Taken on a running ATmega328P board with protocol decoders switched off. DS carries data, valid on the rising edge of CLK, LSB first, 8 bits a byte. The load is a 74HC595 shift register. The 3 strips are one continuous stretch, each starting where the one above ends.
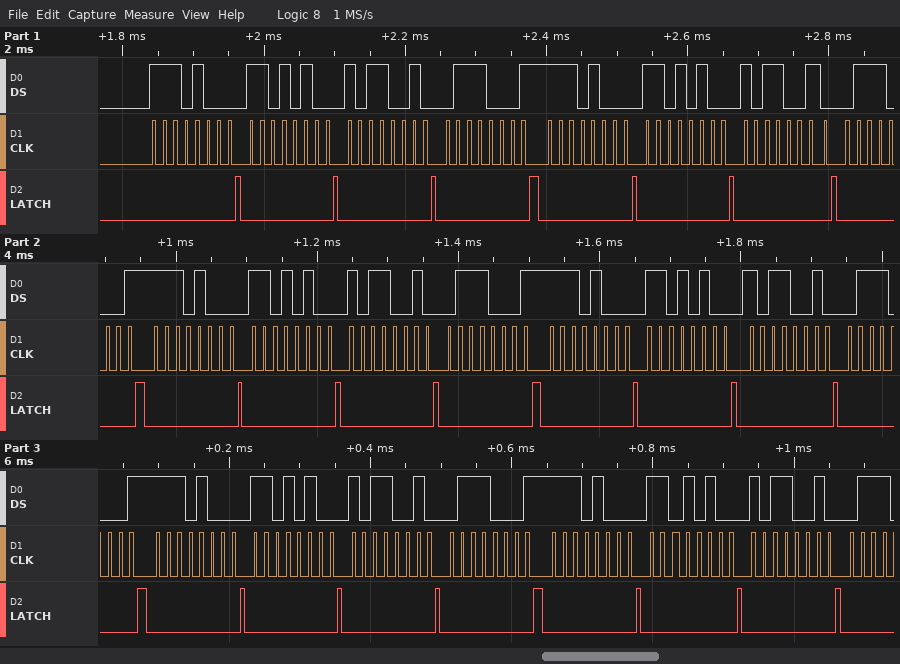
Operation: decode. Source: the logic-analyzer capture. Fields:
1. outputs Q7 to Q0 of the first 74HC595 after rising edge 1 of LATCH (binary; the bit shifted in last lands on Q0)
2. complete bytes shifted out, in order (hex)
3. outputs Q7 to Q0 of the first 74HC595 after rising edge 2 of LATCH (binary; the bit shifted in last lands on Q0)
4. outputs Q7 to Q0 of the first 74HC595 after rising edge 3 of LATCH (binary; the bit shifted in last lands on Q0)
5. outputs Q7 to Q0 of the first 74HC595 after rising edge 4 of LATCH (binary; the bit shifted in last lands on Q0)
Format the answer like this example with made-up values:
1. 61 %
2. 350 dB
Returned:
1. 11101000
2. 0x17 0x2B 0x4D 0x8E 0x17 0x2B 0x4D 0x8E 0x17 0x2B 0x4D 0x8E 0x17 0x2B 0x4D 0x8E 0x17 0x2B 0x4D 0x8E 0x17 0x2B 0x4D
3. 11010100
4. 10110010
5. 01110001
